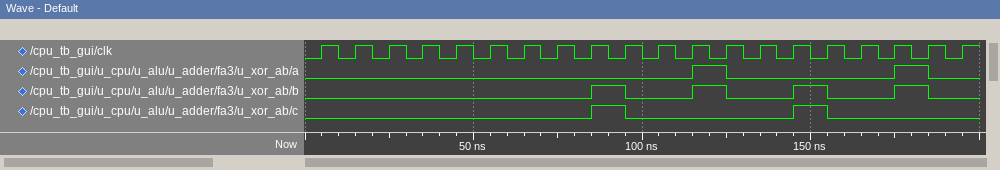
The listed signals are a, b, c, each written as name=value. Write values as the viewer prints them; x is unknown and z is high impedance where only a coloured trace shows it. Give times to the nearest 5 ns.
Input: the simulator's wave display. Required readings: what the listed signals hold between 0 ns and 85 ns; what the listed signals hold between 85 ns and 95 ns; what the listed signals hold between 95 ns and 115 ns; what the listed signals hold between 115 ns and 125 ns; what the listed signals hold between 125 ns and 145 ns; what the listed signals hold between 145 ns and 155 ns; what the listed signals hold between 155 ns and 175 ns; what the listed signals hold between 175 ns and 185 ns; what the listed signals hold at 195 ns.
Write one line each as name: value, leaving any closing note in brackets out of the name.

what the listed signals hold between 0 ns and 85 ns: a=0, b=0, c=0
what the listed signals hold between 85 ns and 95 ns: a=0, b=1, c=1
what the listed signals hold between 95 ns and 115 ns: a=0, b=0, c=0
what the listed signals hold between 115 ns and 125 ns: a=1, b=1, c=0
what the listed signals hold between 125 ns and 145 ns: a=0, b=0, c=0
what the listed signals hold between 145 ns and 155 ns: a=0, b=1, c=1
what the listed signals hold between 155 ns and 175 ns: a=0, b=0, c=0
what the listed signals hold between 175 ns and 185 ns: a=1, b=1, c=0
what the listed signals hold at 195 ns: a=0, b=0, c=0
